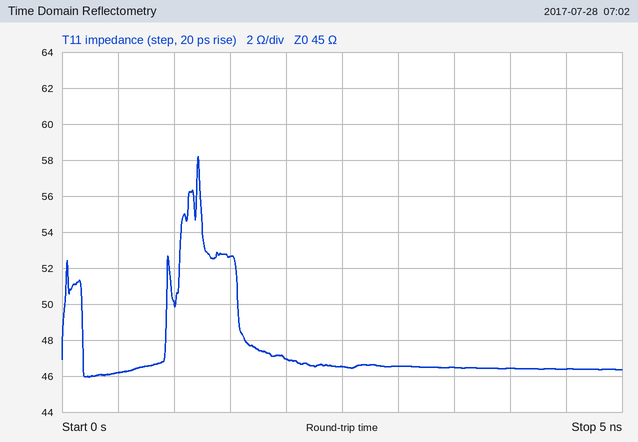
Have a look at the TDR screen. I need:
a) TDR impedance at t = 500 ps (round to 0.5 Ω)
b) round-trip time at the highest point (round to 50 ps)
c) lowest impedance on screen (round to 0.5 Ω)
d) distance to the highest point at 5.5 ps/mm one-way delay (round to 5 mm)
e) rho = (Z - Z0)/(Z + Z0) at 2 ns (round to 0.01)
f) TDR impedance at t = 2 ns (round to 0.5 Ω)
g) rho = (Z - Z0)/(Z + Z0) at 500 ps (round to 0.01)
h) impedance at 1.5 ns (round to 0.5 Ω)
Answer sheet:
46.0 Ω
1.20 ns
46.0 Ω
110 mm
+0.02
47.0 Ω
+0.01
52.5 Ω
